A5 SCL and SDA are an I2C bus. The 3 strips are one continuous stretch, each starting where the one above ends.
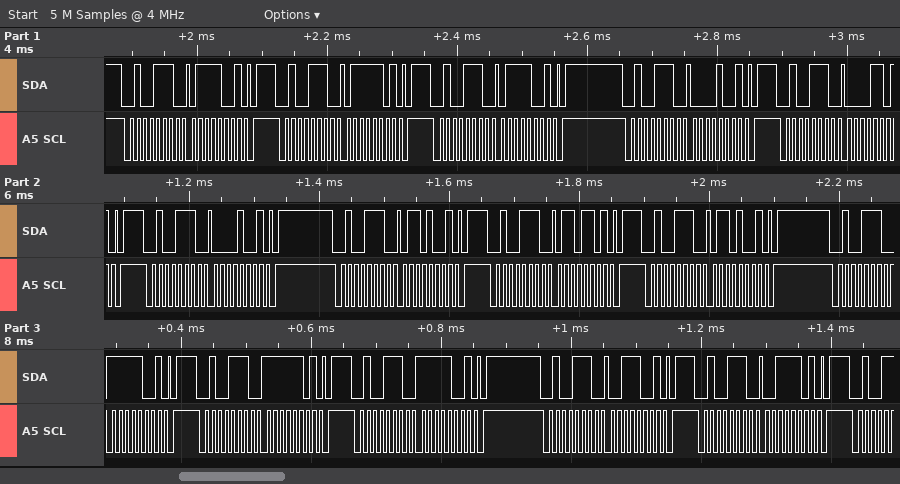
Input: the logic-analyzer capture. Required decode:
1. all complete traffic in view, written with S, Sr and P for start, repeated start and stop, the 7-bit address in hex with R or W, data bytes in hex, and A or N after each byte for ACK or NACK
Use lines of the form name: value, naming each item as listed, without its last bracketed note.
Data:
all complete traffic in view, written with S, Sr and P for start, repeated start and stop, the 7-bit address in hex with R or W, data bytes in hex, and A or N after each byte for ACK or NACK: S 27W A 79 A P S 27W A 7D A P S 27W A 79 A P S 27W A 09 A P S 27W A 0D A P S 27W A 09 A P S 27W A 69 A P S 27W A 6D A P S 27W A 69 A P S 27W A F9 A P S 27W A FD A P S 27W A F9 A P S 27W A 39 A P S 27W A 3D A P
